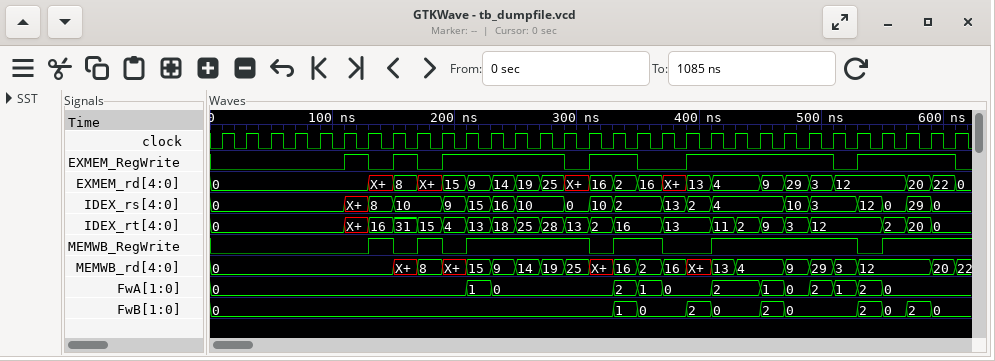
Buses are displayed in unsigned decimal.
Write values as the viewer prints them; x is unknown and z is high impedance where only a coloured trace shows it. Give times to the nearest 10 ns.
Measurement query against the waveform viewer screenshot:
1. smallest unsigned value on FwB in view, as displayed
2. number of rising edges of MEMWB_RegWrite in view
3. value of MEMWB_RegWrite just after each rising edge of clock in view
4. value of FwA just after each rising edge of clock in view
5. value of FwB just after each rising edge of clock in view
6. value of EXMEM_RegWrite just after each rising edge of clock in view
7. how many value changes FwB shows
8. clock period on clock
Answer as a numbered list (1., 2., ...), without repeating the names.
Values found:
1. 0
2. 6
3. 0 0 0 0 0 0 1 0 1 0 1 1 1 1 1 0 1 1 0 0 1 1 1 1 1 1 0 1 1 1 1
4. 0, 0, 0, 0, 0, 0, 0, 0, 0, 0, 1, 0, 0, 0, 0, 0, 2, 1, 0, 0, 2, 2, 1, 0, 2, 1, 2, 0, 0, 0, 0
5. 0, 0, 0, 0, 0, 0, 0, 0, 0, 0, 0, 0, 0, 0, 0, 0, 1, 0, 0, 2, 0, 0, 2, 0, 0, 0, 2, 0, 2, 0, 0
6. 0 0 0 0 0 1 0 1 0 1 1 1 1 1 0 1 1 0 0 1 1 1 1 1 1 0 1 1 1 1 0
7. 10
8. 20 ns
